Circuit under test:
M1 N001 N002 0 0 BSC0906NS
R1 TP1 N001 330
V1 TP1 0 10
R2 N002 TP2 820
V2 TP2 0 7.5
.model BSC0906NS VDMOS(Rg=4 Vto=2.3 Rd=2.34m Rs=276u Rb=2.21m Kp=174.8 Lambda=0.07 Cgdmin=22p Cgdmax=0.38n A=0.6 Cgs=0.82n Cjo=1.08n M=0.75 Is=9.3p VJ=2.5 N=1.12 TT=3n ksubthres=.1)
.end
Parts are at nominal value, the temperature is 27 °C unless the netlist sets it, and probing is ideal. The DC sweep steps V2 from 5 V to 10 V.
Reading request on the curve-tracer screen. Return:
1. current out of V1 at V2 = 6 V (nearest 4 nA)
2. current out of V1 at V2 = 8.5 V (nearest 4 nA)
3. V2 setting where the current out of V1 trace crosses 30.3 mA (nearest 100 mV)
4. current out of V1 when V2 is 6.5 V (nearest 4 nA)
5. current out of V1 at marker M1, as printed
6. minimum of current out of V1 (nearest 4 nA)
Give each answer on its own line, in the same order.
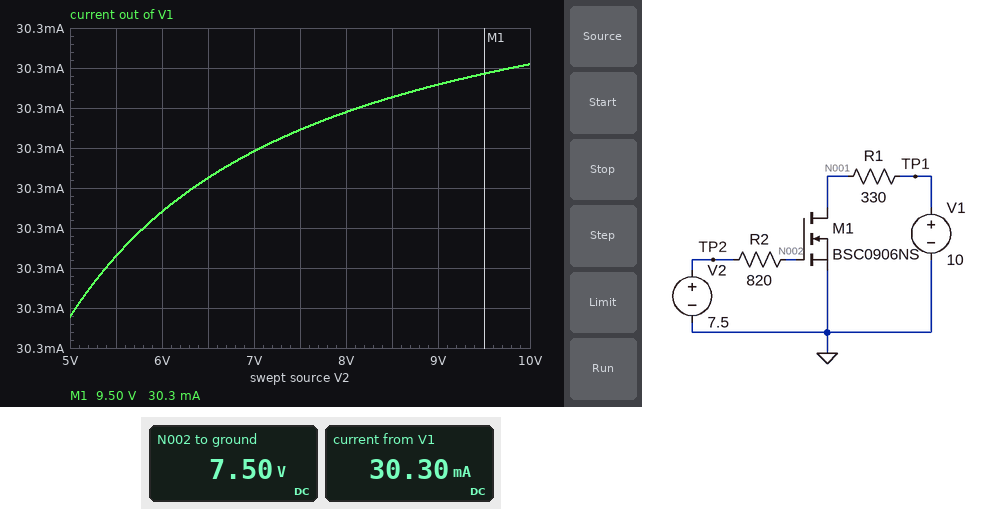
30.302648 mA
30.302704 mA
5.8 V
30.302664 mA
30.3 mA
30.302596 mA
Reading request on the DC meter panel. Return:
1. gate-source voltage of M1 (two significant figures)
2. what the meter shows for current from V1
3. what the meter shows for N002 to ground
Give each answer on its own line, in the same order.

7.5 V
30.30 mA
7.50 V
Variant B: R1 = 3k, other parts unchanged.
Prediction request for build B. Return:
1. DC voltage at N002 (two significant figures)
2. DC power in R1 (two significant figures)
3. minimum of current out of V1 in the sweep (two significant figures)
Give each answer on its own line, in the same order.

7.5 V
33 mW
3.3 mA
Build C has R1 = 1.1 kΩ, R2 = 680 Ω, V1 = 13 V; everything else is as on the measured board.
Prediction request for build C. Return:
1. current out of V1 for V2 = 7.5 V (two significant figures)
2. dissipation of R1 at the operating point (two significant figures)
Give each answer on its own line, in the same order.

12 mA
150 mW
